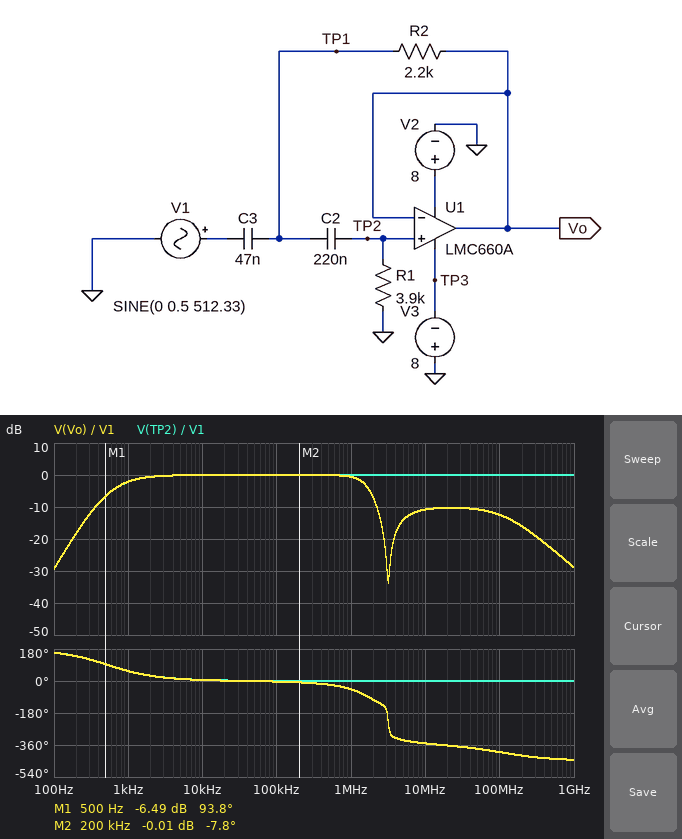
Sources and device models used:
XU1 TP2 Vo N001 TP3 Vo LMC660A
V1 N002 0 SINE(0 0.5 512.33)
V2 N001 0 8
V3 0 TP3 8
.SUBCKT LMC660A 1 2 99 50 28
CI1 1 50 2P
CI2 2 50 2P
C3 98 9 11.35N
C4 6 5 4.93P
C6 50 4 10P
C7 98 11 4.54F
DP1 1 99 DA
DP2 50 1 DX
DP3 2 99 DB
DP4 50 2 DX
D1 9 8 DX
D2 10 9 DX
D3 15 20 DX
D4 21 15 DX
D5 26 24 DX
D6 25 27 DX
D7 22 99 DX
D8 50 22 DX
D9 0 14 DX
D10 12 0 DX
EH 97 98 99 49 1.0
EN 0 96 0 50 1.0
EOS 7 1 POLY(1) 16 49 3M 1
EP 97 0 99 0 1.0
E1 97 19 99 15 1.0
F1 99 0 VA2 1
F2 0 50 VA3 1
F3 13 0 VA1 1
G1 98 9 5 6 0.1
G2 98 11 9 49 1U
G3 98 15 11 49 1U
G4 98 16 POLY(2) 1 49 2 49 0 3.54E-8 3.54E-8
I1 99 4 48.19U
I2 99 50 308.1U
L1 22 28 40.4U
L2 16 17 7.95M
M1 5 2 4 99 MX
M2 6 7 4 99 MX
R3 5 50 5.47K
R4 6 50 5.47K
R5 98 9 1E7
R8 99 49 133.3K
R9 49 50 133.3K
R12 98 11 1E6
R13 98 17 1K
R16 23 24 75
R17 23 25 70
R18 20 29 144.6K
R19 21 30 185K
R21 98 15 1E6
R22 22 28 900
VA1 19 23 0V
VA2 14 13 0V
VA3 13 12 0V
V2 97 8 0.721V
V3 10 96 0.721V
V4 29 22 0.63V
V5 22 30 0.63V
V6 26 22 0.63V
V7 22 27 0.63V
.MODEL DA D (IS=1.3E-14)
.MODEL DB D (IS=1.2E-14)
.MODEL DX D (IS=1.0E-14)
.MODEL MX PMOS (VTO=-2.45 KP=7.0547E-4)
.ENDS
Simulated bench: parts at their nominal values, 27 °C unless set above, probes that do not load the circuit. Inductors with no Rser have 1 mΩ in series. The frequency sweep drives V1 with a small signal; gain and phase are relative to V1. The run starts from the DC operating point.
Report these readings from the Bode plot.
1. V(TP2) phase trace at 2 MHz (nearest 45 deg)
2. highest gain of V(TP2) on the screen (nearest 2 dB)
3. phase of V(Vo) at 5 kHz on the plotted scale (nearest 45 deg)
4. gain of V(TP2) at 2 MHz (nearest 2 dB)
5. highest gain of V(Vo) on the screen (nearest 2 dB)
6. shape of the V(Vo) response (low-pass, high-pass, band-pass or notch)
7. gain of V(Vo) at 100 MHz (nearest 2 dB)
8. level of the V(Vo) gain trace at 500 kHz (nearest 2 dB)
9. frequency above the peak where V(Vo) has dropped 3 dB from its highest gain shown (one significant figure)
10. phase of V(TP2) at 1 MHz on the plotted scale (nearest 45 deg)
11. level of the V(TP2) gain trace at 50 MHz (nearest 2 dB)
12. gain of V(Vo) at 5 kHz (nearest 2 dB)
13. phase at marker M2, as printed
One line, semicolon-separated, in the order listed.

0 deg; 0 dB; 0 deg; 0 dB; 0 dB; band-pass; -12 dB; 0 dB; 2 MHz; 0 deg; 0 dB; 0 dB; -7.8 deg
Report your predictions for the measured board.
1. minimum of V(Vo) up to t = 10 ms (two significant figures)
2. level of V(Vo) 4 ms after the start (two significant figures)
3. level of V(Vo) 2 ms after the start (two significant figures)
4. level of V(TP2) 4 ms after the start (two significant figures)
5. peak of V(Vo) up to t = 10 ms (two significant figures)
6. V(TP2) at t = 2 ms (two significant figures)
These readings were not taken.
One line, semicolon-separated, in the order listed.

-240 mV; 230 mV; 240 mV; 230 mV; 250 mV; 240 mV
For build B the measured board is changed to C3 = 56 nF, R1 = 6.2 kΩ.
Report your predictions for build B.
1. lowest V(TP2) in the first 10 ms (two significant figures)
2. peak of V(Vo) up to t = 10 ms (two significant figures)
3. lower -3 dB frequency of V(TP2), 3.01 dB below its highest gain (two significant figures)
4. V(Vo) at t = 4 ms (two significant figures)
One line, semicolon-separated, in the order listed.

-420 mV; 430 mV; 410 Hz; 420 mV
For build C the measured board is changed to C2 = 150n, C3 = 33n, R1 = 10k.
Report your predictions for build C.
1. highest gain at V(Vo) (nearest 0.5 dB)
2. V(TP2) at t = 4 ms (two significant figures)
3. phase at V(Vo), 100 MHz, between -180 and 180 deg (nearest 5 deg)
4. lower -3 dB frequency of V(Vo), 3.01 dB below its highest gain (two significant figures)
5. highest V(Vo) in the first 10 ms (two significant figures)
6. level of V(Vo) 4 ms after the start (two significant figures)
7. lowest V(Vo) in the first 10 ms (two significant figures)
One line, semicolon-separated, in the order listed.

0.5 dB; 420 mV; -40 deg; 440 Hz; 440 mV; 430 mV; -430 mV
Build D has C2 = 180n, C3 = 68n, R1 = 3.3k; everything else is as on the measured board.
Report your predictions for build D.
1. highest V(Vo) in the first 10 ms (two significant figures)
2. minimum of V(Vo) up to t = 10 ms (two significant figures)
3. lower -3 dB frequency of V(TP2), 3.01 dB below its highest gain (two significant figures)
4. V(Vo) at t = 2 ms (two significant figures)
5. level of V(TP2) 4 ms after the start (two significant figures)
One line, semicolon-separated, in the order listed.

270 mV; -260 mV; 730 Hz; 260 mV; 250 mV
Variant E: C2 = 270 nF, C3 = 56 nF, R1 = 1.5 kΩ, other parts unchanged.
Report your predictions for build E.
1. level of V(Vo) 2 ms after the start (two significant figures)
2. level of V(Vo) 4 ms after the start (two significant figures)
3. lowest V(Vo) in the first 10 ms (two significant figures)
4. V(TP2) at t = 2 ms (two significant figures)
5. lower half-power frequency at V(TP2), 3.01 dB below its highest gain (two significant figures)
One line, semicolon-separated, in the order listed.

110 mV; 98 mV; -110 mV; 100 mV; 2.1 kHz
